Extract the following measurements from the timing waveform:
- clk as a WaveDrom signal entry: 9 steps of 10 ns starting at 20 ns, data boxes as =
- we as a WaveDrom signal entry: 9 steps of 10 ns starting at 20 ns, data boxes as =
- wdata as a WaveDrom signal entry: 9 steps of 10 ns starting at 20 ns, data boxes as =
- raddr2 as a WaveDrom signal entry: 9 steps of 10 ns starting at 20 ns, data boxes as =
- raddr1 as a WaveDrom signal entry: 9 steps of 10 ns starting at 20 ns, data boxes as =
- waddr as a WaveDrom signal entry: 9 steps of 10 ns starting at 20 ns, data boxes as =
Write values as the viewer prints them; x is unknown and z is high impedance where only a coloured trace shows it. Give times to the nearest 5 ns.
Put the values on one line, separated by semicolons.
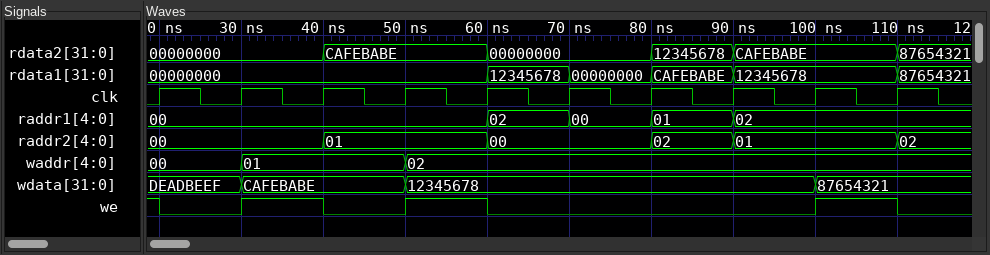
{name: 'clk', wave: 'p........'}; {name: 'we', wave: '01010...1'}; {name: 'wdata', wave: '==.=....=', data: 'DEADBEEF CAFEBABE 12345678 87654321'}; {name: 'raddr2', wave: '=.=.=.==.', data: '00 01 00 02 01'}; {name: 'raddr1', wave: '=...====.', data: '00 02 00 01 02'}; {name: 'waddr', wave: '==.=.....', data: '00 01 02'}
